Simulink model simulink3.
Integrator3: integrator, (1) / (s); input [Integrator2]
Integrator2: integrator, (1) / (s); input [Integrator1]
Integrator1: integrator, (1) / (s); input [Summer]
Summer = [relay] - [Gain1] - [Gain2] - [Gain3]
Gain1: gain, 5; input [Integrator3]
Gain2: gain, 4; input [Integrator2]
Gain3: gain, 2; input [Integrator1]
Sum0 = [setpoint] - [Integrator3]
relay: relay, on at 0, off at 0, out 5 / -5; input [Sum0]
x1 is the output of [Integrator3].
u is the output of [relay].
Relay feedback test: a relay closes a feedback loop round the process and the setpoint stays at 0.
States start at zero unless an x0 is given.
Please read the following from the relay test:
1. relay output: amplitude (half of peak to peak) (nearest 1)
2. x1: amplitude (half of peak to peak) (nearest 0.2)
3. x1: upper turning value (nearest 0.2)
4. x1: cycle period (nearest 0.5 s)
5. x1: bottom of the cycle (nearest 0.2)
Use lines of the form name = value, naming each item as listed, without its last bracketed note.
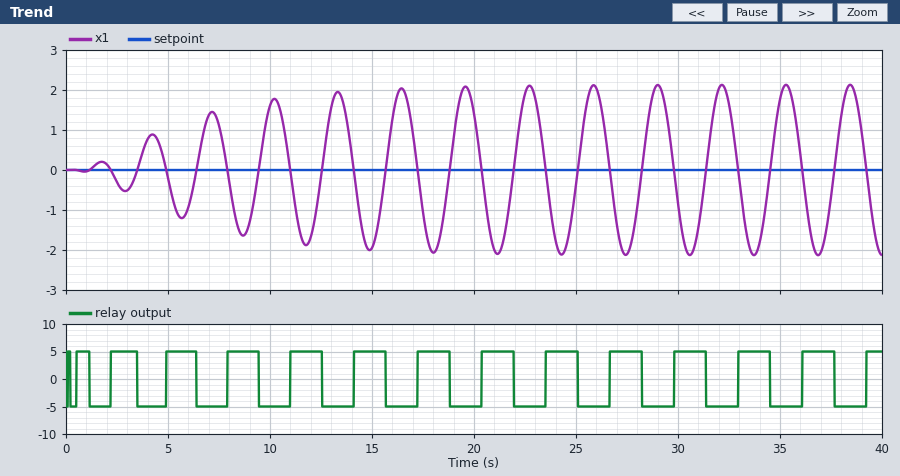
relay output: amplitude (half of peak to peak) = 5
x1: amplitude (half of peak to peak) = 2.2
x1: upper turning value = 2.2
x1: cycle period = 3.0 s
x1: bottom of the cycle = -2.2
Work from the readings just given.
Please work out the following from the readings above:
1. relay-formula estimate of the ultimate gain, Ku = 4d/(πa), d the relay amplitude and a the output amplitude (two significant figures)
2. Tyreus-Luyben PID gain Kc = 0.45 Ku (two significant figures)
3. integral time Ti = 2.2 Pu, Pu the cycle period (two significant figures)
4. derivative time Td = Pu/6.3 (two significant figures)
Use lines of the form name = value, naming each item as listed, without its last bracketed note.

relay-formula estimate of the ultimate gain, Ku = 4d/(πa), d the relay amplitude and a the output amplitude = 2.9
Tyreus-Luyben PID gain Kc = 0.45 Ku = 1.3
integral time Ti = 2.2 Pu, Pu the cycle period = 6.6 s
derivative time Td = Pu/6.3 = 0.48 s
